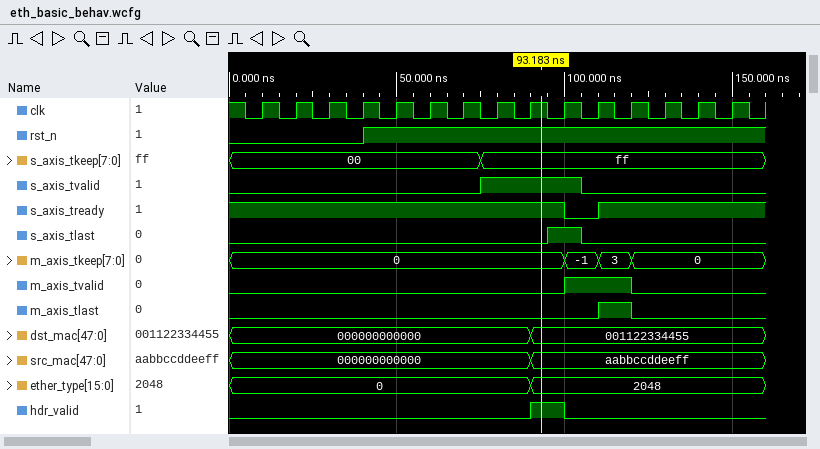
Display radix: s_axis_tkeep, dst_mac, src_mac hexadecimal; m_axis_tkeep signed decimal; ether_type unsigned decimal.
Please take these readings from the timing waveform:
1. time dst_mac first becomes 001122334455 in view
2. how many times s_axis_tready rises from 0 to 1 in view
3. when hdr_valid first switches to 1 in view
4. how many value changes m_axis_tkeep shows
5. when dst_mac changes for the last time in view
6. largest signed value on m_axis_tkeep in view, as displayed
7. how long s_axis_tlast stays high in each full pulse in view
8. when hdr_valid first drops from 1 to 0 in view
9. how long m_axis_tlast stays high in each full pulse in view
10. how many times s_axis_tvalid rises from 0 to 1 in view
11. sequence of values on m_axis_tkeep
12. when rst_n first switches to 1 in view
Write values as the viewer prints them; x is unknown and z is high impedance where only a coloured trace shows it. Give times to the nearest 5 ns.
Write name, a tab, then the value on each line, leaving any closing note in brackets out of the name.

time dst_mac first becomes 001122334455 in view	90 ns
how many times s_axis_tready rises from 0 to 1 in view	1
when hdr_valid first switches to 1 in view	90 ns
how many value changes m_axis_tkeep shows	3
when dst_mac changes for the last time in view	90 ns
largest signed value on m_axis_tkeep in view, as displayed	3
how long s_axis_tlast stays high in each full pulse in view	10 ns
when hdr_valid first drops from 1 to 0 in view	100 ns
how long m_axis_tlast stays high in each full pulse in view	10 ns
how many times s_axis_tvalid rises from 0 to 1 in view	1
sequence of values on m_axis_tkeep	0, -1, 3, 0
when rst_n first switches to 1 in view	40 ns
